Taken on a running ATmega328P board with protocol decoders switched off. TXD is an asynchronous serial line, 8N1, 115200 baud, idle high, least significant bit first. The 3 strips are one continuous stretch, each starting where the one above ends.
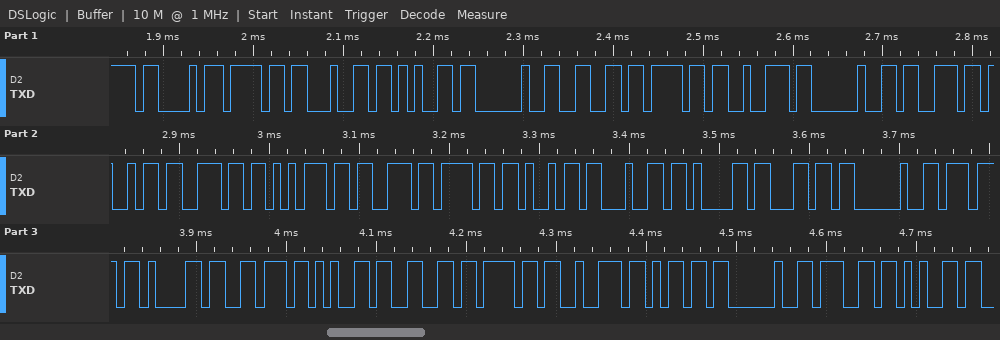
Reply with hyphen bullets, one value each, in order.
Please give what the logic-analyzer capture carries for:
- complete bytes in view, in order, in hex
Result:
- 43 6F 64 65 20 66 6F 72 20 73 69 6E 75 73 6F 69 64 61 6C 20 77 61 76 65 66 6F 72 6D 20 67 65
